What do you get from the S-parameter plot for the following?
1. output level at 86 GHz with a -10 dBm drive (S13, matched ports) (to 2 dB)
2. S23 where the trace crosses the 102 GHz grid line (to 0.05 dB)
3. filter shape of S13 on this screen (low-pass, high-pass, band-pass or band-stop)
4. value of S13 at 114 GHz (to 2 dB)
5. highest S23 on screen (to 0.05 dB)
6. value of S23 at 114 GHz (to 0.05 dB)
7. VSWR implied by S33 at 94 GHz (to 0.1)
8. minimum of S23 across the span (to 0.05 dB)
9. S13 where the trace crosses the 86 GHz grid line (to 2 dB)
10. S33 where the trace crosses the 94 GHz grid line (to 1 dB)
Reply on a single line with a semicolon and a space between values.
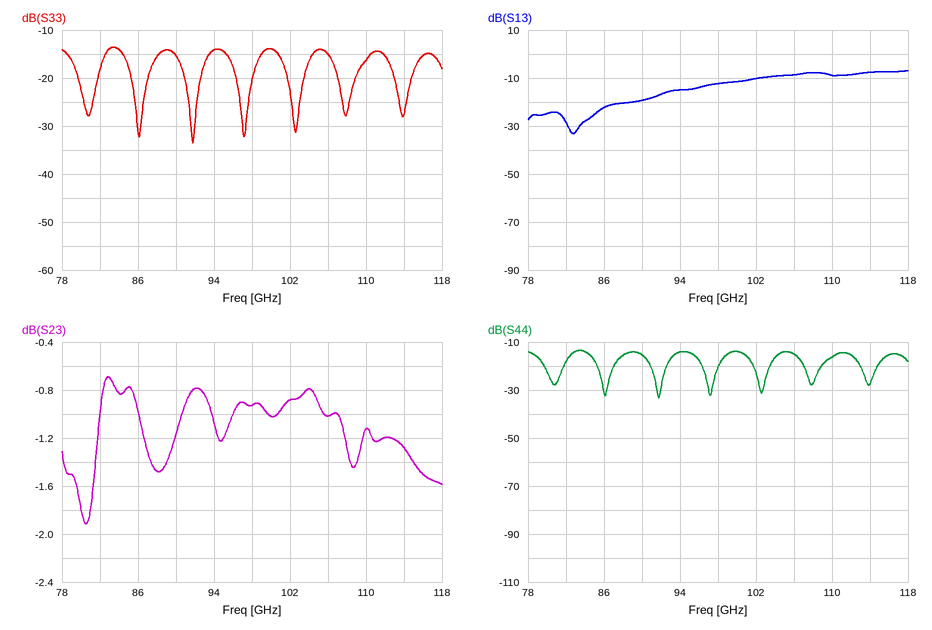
-32 dBm; -0.90 dB; high-pass; -8 dB; -0.70 dB; -1.30 dB; 1.5; -1.90 dB; -22 dB; -14 dB
